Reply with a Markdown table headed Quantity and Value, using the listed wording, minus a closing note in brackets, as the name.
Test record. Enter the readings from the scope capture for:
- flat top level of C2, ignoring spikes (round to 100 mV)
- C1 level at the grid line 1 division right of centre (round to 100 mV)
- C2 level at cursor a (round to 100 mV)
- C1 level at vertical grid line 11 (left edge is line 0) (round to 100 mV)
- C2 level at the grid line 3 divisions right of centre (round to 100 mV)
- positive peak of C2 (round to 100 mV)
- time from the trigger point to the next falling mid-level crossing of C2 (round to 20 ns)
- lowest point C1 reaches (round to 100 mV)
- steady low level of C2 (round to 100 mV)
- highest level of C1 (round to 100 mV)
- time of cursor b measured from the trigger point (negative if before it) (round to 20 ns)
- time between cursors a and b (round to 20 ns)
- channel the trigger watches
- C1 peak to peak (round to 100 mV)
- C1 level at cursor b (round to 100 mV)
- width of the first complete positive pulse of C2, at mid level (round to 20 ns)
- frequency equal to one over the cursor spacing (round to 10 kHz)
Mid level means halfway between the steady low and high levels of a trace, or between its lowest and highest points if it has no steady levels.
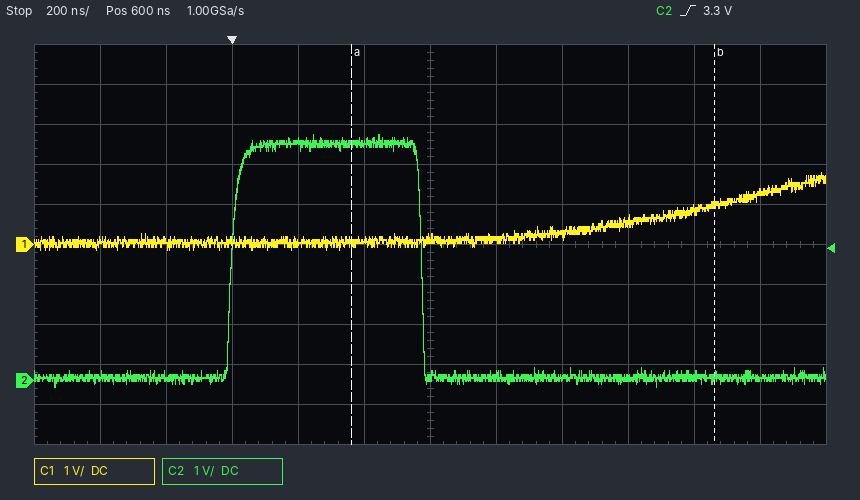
| Quantity | Value |
|---|---|
| flat top level of C2, ignoring spikes | 5.9 V |
| C1 level at the grid line 1 division right of centre | 100 mV |
| C2 level at cursor a | 5.9 V |
| C1 level at vertical grid line 11 (left edge is line 0) | 1.3 V |
| C2 level at the grid line 3 divisions right of centre | 100 mV |
| positive peak of C2 | 6.2 V |
| time from the trigger point to the next falling mid-level crossing of C2 | 580 ns |
| lowest point C1 reaches | -100 mV |
| steady low level of C2 | 100 mV |
| highest level of C1 | 1.8 V |
| time of cursor b measured from the trigger point (negative if before it) | +1.46 µs |
| time between cursors a and b | 1.10 µs |
| channel the trigger watches | C2 |
| C1 peak to peak | 1.9 V |
| C1 level at cursor b | 1.0 V |
| width of the first complete positive pulse of C2, at mid level | 580 ns |
| frequency equal to one over the cursor spacing | 910 kHz |
